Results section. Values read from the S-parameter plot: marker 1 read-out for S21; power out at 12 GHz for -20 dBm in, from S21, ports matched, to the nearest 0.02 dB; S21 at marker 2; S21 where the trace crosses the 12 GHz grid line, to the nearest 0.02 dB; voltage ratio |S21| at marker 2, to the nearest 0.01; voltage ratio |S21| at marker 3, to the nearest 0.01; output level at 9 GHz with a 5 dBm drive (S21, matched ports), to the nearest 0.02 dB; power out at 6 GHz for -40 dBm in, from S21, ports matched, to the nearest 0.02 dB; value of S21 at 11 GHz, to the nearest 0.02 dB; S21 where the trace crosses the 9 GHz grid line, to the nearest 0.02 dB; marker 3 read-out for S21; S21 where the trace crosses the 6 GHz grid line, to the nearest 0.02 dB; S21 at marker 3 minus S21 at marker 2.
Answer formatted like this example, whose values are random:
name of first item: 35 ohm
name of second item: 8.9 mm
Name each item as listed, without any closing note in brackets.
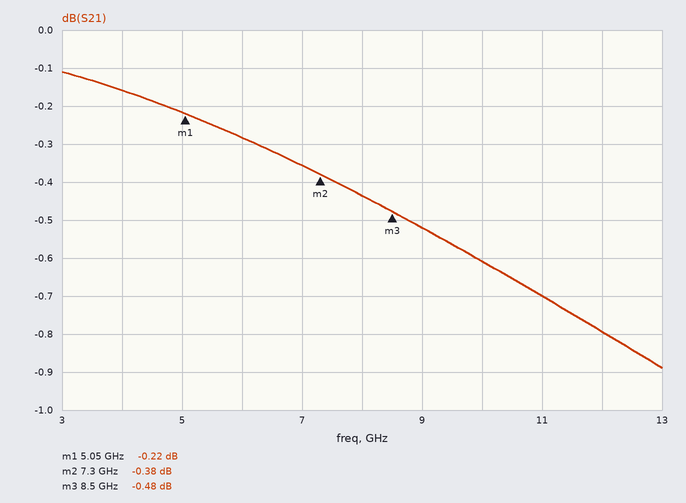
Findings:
marker 1 read-out for S21: -0.22 dB
power out at 12 GHz for -20 dBm in, from S21, ports matched, to the nearest 0.02 dB: -20.80 dBm
S21 at marker 2: -0.38 dB
S21 where the trace crosses the 12 GHz grid line, to the nearest 0.02 dB: -0.80 dB
voltage ratio |S21| at marker 2, to the nearest 0.01: 0.96
voltage ratio |S21| at marker 3, to the nearest 0.01: 0.95
output level at 9 GHz with a 5 dBm drive (S21, matched ports), to the nearest 0.02 dB: 4.48 dBm
power out at 6 GHz for -40 dBm in, from S21, ports matched, to the nearest 0.02 dB: -40.28 dBm
value of S21 at 11 GHz, to the nearest 0.02 dB: -0.70 dB
S21 where the trace crosses the 9 GHz grid line, to the nearest 0.02 dB: -0.52 dB
marker 3 read-out for S21: -0.48 dB
S21 where the trace crosses the 6 GHz grid line, to the nearest 0.02 dB: -0.28 dB
S21 at marker 3 minus S21 at marker 2: -0.10 dB
